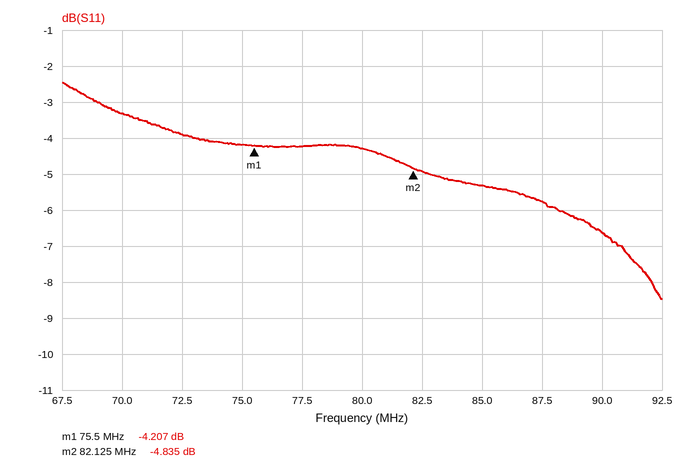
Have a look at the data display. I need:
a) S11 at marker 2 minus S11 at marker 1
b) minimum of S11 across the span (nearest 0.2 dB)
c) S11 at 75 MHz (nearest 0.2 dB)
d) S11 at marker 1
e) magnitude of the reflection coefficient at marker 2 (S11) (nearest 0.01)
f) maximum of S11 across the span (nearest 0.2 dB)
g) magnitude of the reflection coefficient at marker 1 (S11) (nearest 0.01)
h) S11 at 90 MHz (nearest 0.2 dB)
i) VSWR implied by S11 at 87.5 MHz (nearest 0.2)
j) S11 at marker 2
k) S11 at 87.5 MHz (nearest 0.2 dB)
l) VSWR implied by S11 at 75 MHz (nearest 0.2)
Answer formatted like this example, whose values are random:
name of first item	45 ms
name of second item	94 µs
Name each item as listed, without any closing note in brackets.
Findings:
S11 at marker 2 minus S11 at marker 1	-0.628 dB
minimum of S11 across the span	-8.4 dB
S11 at 75 MHz	-4.2 dB
S11 at marker 1	-4.207 dB
magnitude of the reflection coefficient at marker 2 (S11)	0.57
maximum of S11 across the span	-2.4 dB
magnitude of the reflection coefficient at marker 1 (S11)	0.62
S11 at 90 MHz	-6.6 dB
VSWR implied by S11 at 87.5 MHz	3.2
S11 at marker 2	-4.835 dB
S11 at 87.5 MHz	-5.8 dB
VSWR implied by S11 at 75 MHz	4.2
